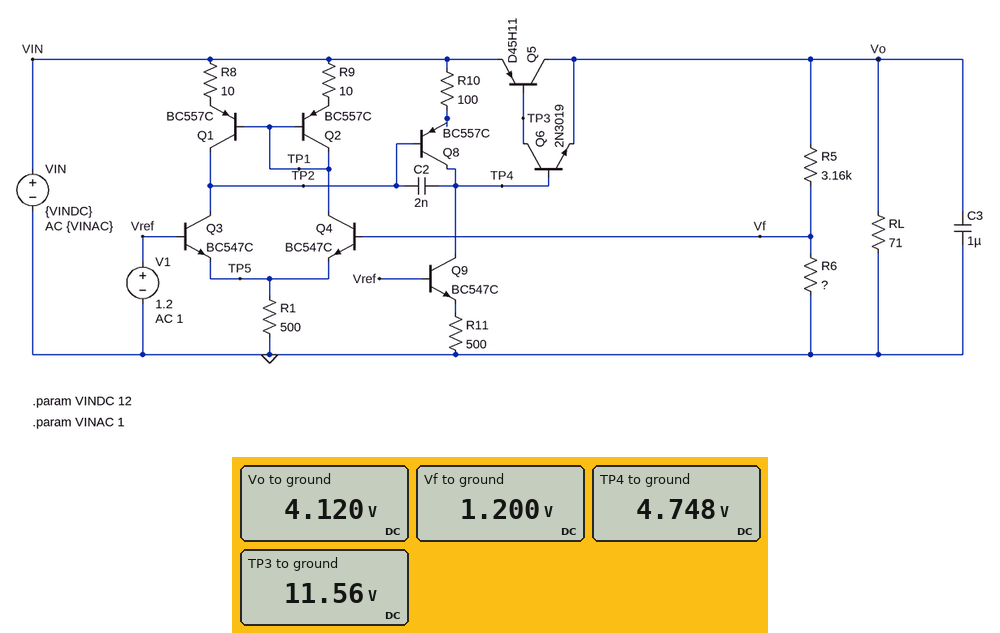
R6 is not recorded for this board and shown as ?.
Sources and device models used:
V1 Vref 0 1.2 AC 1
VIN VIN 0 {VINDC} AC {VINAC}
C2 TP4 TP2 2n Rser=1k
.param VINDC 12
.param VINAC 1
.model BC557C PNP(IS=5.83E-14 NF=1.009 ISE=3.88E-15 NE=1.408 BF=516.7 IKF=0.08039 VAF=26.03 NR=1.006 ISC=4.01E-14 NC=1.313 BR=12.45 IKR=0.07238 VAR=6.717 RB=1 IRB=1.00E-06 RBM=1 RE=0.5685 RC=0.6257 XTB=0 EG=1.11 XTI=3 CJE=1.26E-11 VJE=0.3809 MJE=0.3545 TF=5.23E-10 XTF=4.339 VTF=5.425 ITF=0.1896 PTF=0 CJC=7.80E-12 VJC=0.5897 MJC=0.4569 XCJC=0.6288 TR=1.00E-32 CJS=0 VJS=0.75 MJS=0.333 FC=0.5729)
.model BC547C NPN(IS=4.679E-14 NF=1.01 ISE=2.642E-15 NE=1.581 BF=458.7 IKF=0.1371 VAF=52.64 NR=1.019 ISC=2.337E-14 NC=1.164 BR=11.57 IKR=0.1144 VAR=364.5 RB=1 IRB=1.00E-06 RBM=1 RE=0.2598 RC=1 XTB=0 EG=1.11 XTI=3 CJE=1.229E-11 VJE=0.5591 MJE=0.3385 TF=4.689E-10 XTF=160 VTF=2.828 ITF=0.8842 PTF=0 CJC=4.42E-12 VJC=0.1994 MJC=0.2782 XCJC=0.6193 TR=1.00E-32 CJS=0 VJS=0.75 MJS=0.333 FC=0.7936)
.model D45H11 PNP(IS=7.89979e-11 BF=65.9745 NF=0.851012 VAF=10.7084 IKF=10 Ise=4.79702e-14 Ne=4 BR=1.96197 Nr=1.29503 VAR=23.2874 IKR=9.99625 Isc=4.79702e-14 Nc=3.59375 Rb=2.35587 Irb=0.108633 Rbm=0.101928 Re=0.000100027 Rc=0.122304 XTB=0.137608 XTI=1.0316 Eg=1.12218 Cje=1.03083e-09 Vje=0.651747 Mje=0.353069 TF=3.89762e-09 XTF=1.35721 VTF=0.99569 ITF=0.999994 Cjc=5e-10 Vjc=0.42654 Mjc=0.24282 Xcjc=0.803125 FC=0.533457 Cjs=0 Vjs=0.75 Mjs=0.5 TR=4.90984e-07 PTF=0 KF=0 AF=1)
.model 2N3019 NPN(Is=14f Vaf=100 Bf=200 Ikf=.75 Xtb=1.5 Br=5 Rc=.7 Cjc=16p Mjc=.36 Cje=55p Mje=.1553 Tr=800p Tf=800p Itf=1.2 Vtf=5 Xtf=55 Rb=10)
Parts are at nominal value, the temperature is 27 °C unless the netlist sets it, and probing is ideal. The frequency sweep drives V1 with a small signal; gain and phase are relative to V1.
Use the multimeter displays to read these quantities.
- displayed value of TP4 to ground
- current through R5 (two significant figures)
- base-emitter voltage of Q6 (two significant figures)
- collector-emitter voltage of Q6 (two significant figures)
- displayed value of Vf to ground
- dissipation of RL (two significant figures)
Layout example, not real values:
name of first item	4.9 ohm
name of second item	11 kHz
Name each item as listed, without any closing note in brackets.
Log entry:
displayed value of TP4 to ground	4.748 V
current through R5	920 µA
base-emitter voltage of Q6	630 mV
collector-emitter voltage of Q6	7.4 V
displayed value of Vf to ground	1.200 V
dissipation of RL	240 mW
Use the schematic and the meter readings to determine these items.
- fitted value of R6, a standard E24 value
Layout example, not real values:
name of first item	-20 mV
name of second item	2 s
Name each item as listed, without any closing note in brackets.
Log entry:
fitted value of R6, a standard E24 value	1.3 kΩ
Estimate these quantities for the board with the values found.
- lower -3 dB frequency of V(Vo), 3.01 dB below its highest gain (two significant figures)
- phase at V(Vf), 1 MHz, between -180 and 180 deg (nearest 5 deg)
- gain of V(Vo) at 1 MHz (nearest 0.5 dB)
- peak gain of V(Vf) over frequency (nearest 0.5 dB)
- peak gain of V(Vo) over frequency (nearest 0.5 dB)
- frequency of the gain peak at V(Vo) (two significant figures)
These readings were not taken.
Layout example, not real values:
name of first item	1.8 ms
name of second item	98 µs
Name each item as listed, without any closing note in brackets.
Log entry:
lower -3 dB frequency of V(Vo), 3.01 dB below its highest gain	790 kHz
phase at V(Vf), 1 MHz, between -180 and 180 deg	170 deg
gain of V(Vo) at 1 MHz	17.0 dB
peak gain of V(Vf) over frequency	18.5 dB
peak gain of V(Vo) over frequency	29.5 dB
frequency of the gain peak at V(Vo)	840 kHz
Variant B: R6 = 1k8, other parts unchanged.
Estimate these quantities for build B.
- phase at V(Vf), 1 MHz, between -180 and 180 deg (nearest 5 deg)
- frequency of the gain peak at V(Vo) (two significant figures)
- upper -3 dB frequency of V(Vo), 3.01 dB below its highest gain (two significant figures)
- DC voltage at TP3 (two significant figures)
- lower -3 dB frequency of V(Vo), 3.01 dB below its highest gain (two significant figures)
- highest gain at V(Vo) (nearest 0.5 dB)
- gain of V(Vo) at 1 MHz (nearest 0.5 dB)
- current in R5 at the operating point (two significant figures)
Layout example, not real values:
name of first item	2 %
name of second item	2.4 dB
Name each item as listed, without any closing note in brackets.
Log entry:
phase at V(Vf), 1 MHz, between -180 and 180 deg	160 deg
frequency of the gain peak at V(Vo)	790 kHz
upper -3 dB frequency of V(Vo), 3.01 dB below its highest gain	820 kHz
DC voltage at TP3	12 V
lower -3 dB frequency of V(Vo), 3.01 dB below its highest gain	760 kHz
highest gain at V(Vo)	31.0 dB
gain of V(Vo) at 1 MHz	12.5 dB
current in R5 at the operating point	670 µA
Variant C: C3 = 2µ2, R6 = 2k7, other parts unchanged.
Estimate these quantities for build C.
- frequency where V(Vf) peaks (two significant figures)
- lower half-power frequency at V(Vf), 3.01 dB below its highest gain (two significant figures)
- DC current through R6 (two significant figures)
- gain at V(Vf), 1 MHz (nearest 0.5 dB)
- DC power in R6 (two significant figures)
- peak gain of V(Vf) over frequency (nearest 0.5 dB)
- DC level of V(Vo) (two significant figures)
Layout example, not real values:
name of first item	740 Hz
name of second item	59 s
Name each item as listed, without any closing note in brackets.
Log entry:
frequency where V(Vf) peaks	490 kHz
lower half-power frequency at V(Vf), 3.01 dB below its highest gain	430 kHz
DC current through R6	440 µA
gain at V(Vf), 1 MHz	-9.0 dB
DC power in R6	530 µW
peak gain of V(Vf) over frequency	12.5 dB
DC level of V(Vo)	2.6 V
